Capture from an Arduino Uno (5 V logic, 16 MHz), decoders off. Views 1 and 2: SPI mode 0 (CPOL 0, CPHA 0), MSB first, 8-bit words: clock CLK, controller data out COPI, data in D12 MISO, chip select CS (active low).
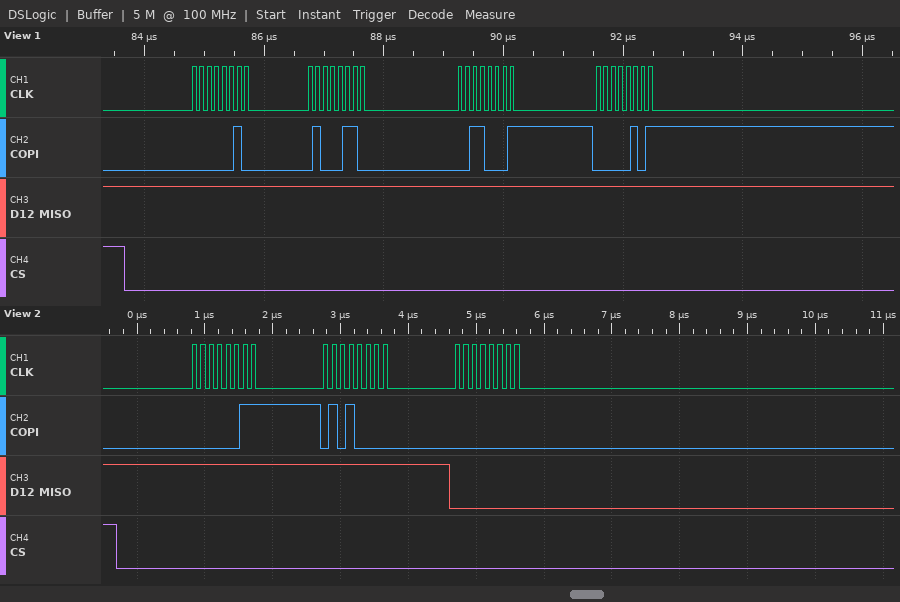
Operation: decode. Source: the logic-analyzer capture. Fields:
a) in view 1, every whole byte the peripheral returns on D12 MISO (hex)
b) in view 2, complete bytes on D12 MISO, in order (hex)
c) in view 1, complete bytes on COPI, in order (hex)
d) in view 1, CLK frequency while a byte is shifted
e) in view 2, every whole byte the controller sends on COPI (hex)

FF FF FF FF
FF FF 00
02 46 31 05
8 MHz
03 50 00
